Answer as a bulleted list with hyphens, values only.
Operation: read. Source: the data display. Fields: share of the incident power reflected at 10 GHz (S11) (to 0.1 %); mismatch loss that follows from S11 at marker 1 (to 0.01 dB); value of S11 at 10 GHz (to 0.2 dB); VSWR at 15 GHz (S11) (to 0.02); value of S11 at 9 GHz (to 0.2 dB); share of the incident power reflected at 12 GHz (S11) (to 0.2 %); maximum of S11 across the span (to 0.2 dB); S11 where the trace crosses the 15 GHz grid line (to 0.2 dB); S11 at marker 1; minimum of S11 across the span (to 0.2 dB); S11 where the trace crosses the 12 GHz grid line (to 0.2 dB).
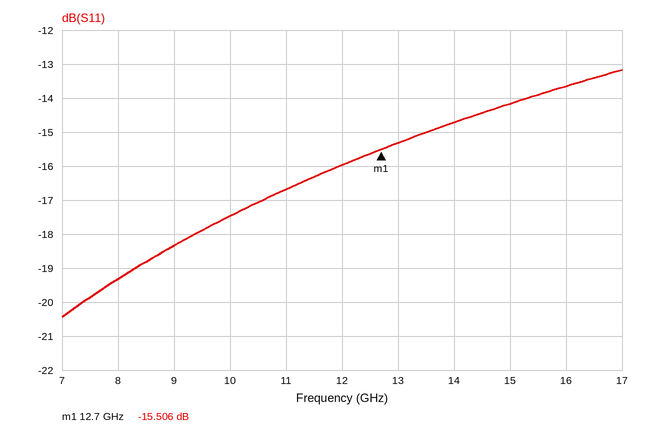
- 1.8 %
- 0.12 dB
- -17.4 dB
- 1.48
- -18.4 dB
- 2.6 %
- -13.2 dB
- -14.2 dB
- -15.506 dB
- -20.4 dB
- -16.0 dB
